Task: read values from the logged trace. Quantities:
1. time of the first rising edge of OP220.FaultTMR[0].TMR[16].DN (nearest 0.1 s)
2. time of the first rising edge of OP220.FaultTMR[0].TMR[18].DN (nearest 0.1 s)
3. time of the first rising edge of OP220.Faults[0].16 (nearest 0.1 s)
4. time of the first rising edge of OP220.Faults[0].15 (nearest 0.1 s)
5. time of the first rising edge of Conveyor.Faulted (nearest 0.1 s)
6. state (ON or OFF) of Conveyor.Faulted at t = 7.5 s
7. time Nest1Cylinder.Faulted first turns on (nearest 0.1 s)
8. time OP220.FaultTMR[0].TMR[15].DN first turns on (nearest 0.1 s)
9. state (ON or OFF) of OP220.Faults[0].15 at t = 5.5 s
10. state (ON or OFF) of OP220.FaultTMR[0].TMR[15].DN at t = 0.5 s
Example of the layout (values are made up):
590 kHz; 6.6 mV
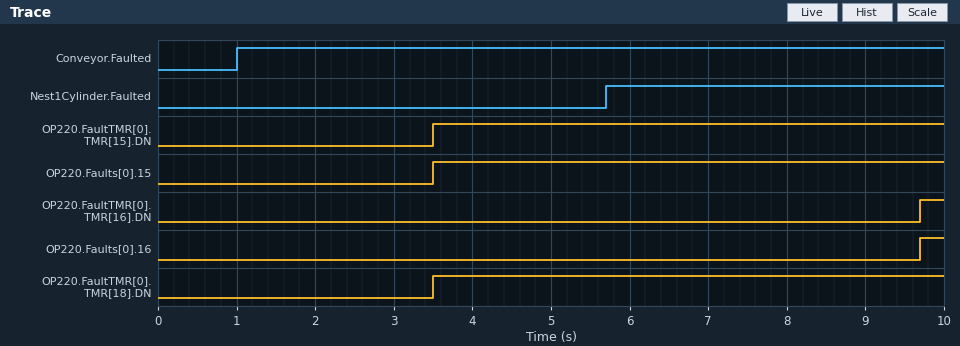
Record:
9.7 s; 3.5 s; 9.7 s; 3.5 s; 1.0 s; ON; 5.7 s; 3.5 s; ON; OFF
